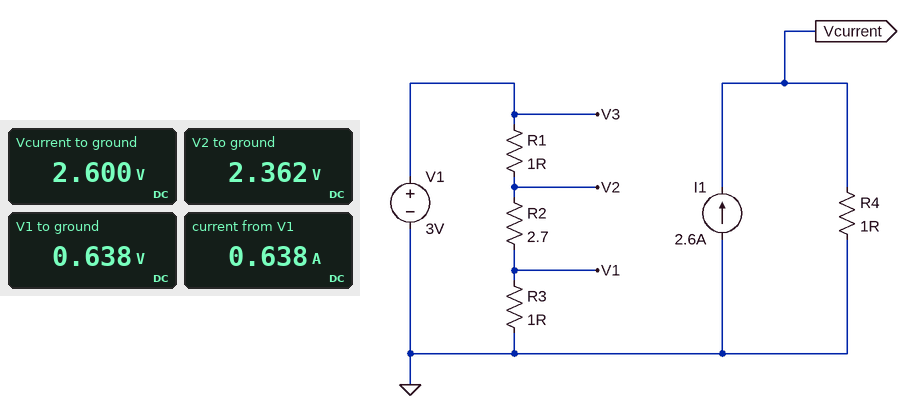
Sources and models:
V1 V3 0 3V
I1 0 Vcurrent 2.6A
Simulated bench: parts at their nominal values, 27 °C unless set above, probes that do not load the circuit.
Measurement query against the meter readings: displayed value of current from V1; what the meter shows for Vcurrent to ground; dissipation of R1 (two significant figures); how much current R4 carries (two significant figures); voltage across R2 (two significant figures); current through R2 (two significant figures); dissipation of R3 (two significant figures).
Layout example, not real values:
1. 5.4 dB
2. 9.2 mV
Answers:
1. 0.638 A
2. 2.600 V
3. 410 mW
4. 2.6 A
5. 1.7 V
6. 640 mA
7. 410 mW
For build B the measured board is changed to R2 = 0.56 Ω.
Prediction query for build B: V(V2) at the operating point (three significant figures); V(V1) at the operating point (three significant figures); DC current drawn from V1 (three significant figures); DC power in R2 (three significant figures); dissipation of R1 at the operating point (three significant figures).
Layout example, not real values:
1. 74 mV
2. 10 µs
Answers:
1. 1.83 V
2. 1.17 V
3. 1.17 A
4. 769 mW
5. 1.37 W
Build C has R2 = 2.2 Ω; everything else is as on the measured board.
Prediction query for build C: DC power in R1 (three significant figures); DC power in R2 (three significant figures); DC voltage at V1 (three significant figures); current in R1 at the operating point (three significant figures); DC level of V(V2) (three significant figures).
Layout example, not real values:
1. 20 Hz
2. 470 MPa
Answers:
1. 510 mW
2. 1.12 W
3. 714 mV
4. 714 mA
5. 2.29 V
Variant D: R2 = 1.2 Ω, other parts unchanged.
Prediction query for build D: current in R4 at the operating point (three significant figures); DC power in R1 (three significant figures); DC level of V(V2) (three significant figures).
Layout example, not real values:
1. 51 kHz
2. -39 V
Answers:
1. 2.60 A
2. 879 mW
3. 2.06 V
